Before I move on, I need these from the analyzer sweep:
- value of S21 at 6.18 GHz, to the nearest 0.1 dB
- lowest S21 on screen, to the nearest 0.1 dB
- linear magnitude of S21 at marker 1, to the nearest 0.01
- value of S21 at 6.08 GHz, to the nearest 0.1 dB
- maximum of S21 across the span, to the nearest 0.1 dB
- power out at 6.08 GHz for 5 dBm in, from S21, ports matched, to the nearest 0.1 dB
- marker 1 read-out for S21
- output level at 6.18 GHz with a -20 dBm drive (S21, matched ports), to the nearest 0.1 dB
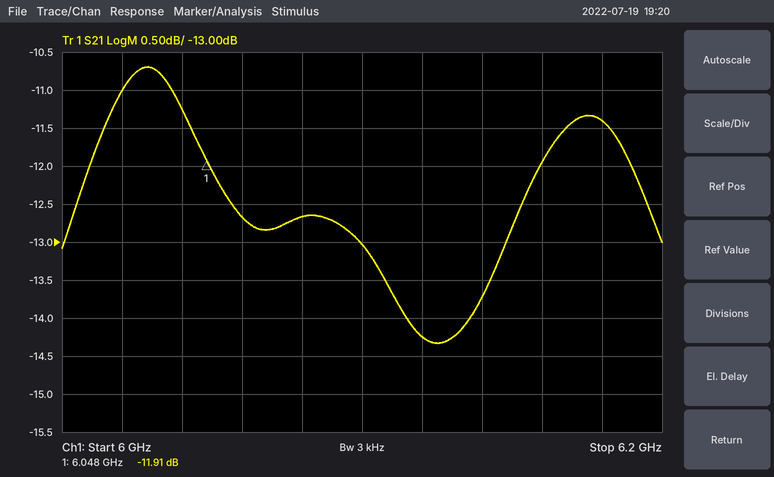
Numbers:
-11.4 dB
-14.3 dB
0.25
-12.7 dB
-10.7 dB
-7.7 dBm
-11.91 dB
-31.4 dBm
